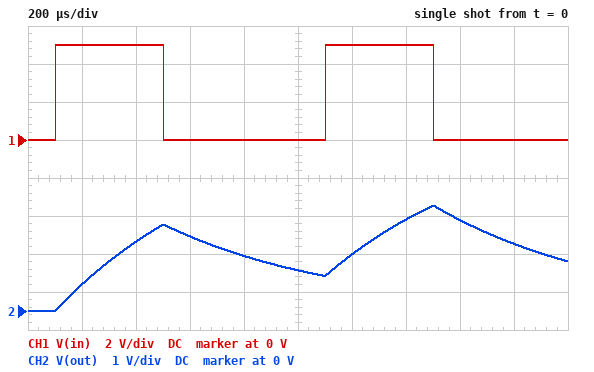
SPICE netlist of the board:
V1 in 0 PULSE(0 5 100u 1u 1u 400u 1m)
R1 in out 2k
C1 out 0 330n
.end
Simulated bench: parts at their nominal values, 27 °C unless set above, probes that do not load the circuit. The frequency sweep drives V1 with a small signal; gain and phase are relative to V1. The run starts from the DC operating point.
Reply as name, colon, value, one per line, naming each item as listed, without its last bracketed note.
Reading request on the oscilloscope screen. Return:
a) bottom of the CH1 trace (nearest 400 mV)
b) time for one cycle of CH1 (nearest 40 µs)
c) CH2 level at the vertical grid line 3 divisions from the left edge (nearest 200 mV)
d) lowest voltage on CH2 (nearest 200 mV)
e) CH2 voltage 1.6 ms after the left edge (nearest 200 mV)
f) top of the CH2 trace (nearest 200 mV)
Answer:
bottom of the CH1 trace: 0 V
time for one cycle of CH1: 1.00 ms
CH2 level at the vertical grid line 3 divisions from the left edge: 2.0 V
lowest voltage on CH2: 0 V
CH2 voltage 1.6 ms after the left edge: 2.4 V
top of the CH2 trace: 2.8 V
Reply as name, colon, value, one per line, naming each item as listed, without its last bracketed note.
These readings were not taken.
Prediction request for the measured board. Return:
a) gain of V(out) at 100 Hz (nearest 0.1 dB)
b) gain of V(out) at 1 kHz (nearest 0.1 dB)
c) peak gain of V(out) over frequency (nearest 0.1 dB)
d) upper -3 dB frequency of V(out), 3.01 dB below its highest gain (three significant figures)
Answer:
gain of V(out) at 100 Hz: -0.7 dB
gain of V(out) at 1 kHz: -12.6 dB
peak gain of V(out) over frequency: 0 dB
upper -3 dB frequency of V(out), 3.01 dB below its highest gain: 241 Hz
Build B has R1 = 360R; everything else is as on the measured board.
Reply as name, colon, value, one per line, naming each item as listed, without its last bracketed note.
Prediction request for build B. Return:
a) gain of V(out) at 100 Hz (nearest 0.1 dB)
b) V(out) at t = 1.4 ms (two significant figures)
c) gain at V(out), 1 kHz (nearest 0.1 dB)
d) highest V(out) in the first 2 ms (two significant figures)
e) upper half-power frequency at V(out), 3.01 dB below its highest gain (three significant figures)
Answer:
gain of V(out) at 100 Hz: 0 dB
V(out) at t = 1.4 ms: 4.6 V
gain at V(out), 1 kHz: -1.9 dB
highest V(out) in the first 2 ms: 4.8 V
upper half-power frequency at V(out), 3.01 dB below its highest gain: 1.34 kHz
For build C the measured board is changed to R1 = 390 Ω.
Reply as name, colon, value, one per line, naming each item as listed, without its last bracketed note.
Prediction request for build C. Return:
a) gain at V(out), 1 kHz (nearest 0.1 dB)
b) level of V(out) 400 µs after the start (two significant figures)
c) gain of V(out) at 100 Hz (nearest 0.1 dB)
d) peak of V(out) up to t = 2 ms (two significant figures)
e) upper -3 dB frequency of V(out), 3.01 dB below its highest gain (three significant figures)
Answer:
gain at V(out), 1 kHz: -2.2 dB
level of V(out) 400 µs after the start: 4.5 V
gain of V(out) at 100 Hz: 0 dB
peak of V(out) up to t = 2 ms: 4.8 V
upper -3 dB frequency of V(out), 3.01 dB below its highest gain: 1.24 kHz
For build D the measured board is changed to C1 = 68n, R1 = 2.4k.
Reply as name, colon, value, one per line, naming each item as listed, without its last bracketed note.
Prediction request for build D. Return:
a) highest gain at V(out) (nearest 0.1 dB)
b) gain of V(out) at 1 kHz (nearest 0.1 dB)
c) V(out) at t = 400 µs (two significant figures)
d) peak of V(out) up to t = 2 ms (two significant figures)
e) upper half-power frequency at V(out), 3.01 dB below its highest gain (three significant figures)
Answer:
highest gain at V(out): 0 dB
gain of V(out) at 1 kHz: -3.1 dB
V(out) at t = 400 µs: 4.2 V
peak of V(out) up to t = 2 ms: 4.6 V
upper half-power frequency at V(out), 3.01 dB below its highest gain: 975 Hz
